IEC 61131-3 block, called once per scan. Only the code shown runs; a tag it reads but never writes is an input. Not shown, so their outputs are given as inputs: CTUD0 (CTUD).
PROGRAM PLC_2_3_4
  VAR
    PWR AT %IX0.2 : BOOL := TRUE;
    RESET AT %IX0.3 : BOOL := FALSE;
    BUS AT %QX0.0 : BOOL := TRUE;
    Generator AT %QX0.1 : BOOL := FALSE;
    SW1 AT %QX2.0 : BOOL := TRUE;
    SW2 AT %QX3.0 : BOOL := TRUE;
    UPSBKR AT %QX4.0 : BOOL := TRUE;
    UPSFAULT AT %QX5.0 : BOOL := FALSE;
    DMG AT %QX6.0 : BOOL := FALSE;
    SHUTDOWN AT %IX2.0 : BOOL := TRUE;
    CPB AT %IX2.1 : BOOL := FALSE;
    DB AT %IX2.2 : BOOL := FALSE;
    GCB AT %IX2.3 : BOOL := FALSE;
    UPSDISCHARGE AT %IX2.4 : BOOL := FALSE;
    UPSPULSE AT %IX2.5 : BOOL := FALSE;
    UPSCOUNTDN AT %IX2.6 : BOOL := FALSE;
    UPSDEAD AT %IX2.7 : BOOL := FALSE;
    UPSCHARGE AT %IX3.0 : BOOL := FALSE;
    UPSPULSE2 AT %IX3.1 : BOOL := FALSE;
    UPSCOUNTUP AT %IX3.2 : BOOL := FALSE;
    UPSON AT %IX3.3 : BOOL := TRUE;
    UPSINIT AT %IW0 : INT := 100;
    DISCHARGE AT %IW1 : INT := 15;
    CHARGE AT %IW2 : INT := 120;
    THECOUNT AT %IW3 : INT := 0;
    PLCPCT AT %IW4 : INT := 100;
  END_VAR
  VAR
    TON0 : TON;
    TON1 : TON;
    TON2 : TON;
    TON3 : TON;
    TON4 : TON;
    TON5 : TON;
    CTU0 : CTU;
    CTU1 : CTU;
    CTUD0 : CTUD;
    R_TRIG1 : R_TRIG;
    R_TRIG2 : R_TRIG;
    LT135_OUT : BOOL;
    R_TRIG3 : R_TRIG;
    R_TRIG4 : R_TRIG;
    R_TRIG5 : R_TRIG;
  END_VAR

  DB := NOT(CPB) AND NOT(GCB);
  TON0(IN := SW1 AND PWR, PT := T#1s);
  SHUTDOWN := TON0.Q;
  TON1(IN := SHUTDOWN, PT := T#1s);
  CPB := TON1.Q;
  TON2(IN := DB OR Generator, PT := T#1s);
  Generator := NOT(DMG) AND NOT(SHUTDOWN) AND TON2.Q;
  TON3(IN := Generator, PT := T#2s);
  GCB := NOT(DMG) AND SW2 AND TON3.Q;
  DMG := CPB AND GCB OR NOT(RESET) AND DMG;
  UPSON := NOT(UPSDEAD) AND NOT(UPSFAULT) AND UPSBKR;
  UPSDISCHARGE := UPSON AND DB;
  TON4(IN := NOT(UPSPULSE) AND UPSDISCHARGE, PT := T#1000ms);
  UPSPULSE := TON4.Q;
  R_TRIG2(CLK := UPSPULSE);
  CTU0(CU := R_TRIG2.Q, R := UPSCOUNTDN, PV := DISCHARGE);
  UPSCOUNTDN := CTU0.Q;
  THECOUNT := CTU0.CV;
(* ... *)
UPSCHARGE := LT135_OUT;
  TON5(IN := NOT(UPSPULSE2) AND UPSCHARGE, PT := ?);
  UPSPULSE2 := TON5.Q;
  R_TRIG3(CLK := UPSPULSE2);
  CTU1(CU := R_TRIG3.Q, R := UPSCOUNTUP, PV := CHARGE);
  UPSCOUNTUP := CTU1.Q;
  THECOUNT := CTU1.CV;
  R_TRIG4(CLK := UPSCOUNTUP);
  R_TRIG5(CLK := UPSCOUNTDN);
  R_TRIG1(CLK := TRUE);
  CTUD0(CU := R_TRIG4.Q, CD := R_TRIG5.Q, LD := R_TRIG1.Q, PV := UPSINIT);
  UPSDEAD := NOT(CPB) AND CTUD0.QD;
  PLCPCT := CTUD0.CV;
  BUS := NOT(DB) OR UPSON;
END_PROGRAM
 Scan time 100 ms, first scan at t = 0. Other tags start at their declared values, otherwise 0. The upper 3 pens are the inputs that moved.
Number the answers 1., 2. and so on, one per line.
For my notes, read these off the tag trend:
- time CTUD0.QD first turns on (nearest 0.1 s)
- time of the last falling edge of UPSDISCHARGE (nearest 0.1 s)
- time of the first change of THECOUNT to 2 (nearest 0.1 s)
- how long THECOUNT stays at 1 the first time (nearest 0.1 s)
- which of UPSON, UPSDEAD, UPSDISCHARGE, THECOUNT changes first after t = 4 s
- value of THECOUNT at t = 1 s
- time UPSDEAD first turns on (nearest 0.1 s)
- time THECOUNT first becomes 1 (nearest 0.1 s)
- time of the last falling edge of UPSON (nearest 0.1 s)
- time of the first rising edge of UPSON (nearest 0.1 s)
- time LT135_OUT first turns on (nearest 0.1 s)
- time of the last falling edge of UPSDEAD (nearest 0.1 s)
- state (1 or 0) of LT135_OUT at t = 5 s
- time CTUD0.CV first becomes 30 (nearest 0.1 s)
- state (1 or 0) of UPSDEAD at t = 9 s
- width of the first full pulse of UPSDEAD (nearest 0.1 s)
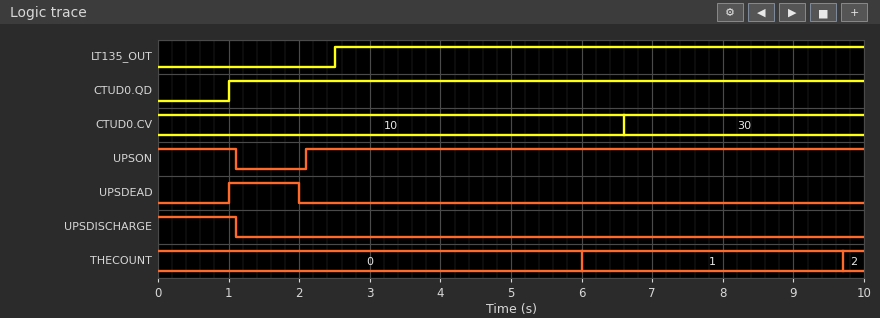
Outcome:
1. 1.0 s
2. 1.1 s
3. 9.7 s
4. 3.7 s
5. THECOUNT
6. 0
7. 1.0 s
8. 6.0 s
9. 1.1 s
10. 2.1 s
11. 2.5 s
12. 2.0 s
13. 1
14. 6.6 s
15. 0
16. 1.0 s
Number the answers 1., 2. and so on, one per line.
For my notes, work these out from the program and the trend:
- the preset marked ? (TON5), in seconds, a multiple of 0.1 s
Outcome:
1. 3.5 s
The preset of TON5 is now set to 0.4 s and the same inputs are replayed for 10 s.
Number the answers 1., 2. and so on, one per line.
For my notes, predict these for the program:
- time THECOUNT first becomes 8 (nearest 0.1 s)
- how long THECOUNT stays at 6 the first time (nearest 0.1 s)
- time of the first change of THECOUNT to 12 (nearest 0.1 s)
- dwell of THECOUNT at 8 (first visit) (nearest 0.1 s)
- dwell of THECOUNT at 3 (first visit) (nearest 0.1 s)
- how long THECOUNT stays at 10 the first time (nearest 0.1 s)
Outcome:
1. 7.1 s
2. 0.6 s
3. 9.5 s
4. 0.6 s
5. 0.6 s
6. 0.6 s
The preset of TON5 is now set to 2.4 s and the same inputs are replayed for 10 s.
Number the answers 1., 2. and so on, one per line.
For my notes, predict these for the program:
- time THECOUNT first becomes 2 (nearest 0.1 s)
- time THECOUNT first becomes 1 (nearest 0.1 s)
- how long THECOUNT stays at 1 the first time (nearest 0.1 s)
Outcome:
1. 7.5 s
2. 4.9 s
3. 2.6 s
